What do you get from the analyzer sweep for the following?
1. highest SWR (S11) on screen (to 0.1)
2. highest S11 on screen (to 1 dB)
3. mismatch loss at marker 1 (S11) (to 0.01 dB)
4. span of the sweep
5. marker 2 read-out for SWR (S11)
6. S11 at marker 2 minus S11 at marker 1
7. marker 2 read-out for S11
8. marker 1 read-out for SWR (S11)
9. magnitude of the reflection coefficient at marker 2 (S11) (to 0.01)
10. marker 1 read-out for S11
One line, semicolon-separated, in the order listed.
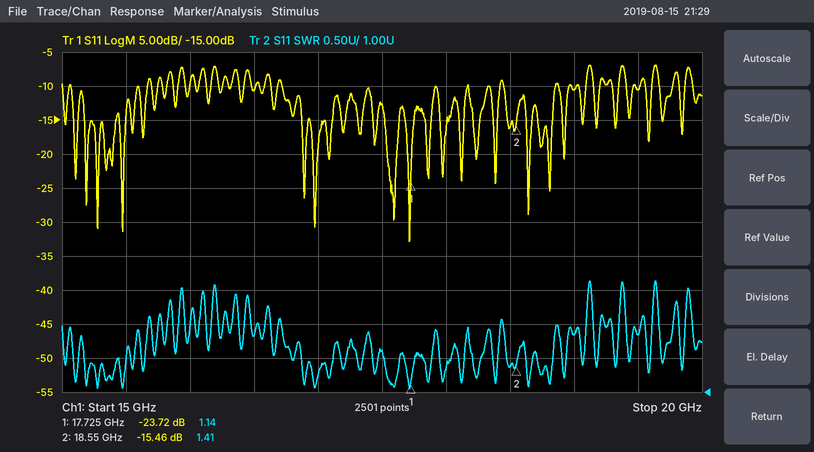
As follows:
2.6; -7 dB; 0.02 dB; 5 GHz; 1.41; 8.26 dB; -15.46 dB; 1.14; 0.17; -23.72 dB
